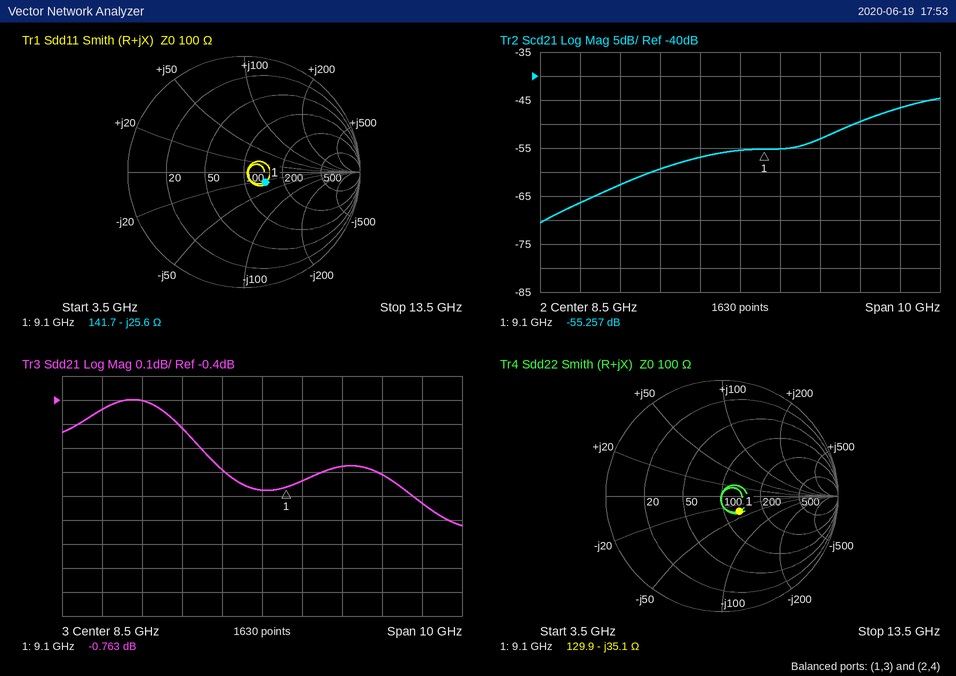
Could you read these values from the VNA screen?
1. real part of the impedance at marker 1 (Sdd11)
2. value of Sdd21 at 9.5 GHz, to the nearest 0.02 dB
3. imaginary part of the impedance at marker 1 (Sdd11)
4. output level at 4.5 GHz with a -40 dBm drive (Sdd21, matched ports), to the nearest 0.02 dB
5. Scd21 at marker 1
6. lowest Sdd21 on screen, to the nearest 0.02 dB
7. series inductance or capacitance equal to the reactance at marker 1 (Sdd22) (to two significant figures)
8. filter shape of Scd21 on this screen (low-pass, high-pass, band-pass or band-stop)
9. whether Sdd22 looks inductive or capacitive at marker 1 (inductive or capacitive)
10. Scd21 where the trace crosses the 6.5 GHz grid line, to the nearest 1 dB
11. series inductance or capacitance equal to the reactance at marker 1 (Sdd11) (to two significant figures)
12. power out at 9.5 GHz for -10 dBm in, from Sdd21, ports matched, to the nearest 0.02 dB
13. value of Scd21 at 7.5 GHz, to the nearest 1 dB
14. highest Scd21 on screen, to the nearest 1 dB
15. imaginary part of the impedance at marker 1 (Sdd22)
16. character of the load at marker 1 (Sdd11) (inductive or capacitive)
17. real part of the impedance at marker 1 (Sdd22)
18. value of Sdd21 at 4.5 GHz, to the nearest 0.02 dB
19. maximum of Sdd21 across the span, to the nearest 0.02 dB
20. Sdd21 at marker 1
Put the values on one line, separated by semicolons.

141.7 Ω; -0.74 dB; -25.6 Ω; -40.44 dBm; -55.257 dB; -0.92 dB; 500 fF; high-pass; capacitive; -59 dB; 680 fF; -10.74 dBm; -57 dB; -45 dB; -35.1 Ω; capacitive; 129.9 Ω; -0.44 dB; -0.40 dB; -0.763 dB
